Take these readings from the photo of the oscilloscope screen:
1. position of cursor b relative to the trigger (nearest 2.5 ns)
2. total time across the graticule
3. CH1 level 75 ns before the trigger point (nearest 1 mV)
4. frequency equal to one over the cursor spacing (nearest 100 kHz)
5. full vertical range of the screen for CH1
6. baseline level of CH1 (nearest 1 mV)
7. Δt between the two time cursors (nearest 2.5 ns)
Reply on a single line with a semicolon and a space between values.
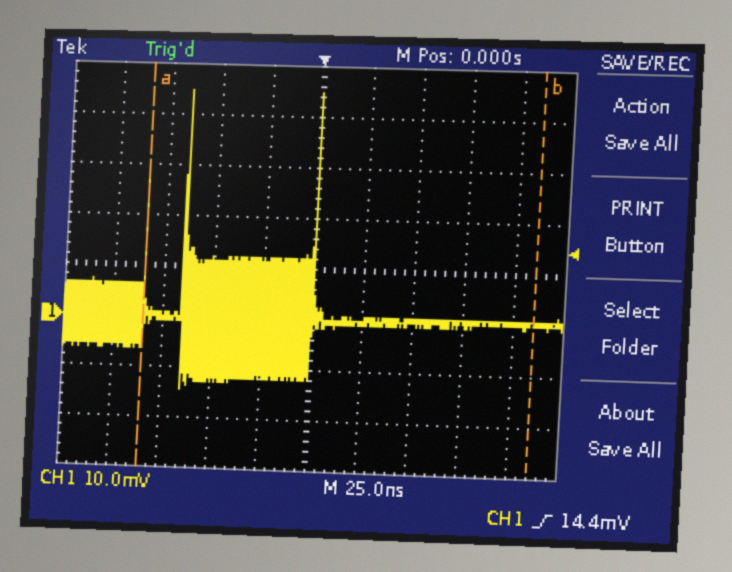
+110.0 ns; 250 ns; 0 mV; 5.1 MHz; 80 mV; 0 mV; 195.0 ns
